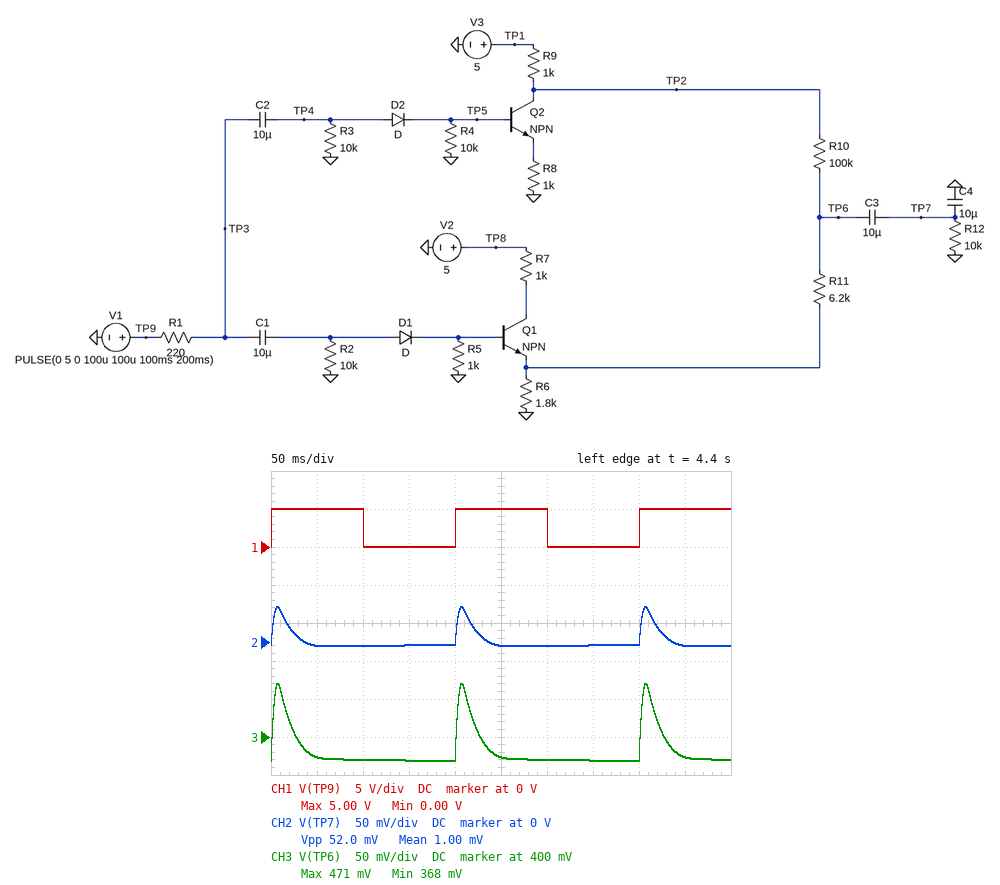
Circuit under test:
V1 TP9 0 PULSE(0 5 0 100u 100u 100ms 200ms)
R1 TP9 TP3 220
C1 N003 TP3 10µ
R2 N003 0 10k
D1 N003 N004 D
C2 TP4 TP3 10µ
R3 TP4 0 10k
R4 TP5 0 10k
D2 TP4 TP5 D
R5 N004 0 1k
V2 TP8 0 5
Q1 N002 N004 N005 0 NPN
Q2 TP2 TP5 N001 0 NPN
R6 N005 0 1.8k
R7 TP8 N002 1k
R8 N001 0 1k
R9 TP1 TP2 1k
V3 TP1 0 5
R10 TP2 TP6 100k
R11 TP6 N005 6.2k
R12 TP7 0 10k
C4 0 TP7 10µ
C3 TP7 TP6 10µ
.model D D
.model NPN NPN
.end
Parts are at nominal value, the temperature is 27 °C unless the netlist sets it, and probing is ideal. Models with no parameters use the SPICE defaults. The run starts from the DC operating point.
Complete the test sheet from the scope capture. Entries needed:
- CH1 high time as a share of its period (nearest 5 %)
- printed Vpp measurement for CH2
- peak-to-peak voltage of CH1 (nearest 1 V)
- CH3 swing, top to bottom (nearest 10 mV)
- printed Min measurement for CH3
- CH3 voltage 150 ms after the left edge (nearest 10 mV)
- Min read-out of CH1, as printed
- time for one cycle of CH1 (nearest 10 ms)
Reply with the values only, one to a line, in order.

50 %
52.0 mV
5 V
100 mV
368 mV
370 mV
0.00 V
200 ms
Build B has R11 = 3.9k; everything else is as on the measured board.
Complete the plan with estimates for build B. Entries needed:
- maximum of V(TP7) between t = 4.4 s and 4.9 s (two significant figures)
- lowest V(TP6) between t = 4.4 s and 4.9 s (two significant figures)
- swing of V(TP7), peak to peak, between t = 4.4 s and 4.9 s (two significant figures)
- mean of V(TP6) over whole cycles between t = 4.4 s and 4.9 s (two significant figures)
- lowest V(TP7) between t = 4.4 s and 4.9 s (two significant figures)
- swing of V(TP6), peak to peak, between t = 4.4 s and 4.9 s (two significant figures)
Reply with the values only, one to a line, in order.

71 mV
270 mV
80 mV
290 mV
-8.7 mV
160 mV
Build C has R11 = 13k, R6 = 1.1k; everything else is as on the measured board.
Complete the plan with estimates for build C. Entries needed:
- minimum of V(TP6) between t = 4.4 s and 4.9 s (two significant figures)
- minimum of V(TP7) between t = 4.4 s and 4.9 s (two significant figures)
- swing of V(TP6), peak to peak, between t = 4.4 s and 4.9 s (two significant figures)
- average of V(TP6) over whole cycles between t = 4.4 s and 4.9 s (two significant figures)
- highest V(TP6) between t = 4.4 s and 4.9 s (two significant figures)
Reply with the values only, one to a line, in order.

600 mV
-6.0 mV
56 mV
610 mV
660 mV
